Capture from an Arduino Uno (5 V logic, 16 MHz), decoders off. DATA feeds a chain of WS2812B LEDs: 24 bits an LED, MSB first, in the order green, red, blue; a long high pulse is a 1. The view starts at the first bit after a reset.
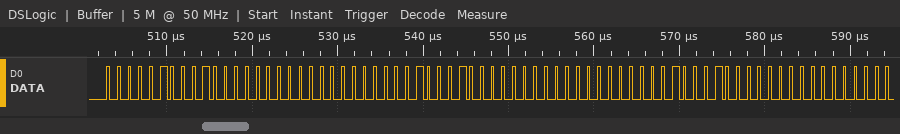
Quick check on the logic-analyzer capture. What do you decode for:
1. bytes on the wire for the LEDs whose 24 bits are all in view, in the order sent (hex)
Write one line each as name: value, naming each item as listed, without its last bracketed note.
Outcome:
bytes on the wire for the LEDs whose 24 bits are all in view, in the order sent: 04 40 00 04 40 00 04 40 00
